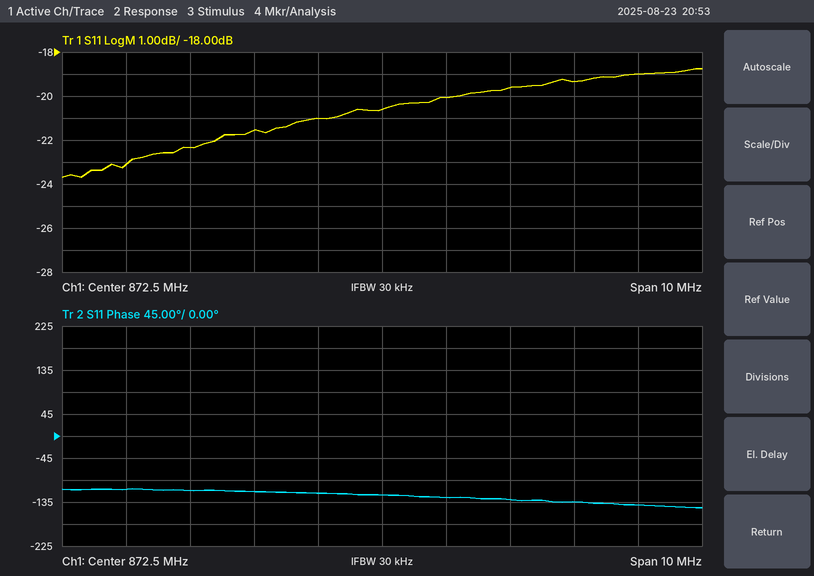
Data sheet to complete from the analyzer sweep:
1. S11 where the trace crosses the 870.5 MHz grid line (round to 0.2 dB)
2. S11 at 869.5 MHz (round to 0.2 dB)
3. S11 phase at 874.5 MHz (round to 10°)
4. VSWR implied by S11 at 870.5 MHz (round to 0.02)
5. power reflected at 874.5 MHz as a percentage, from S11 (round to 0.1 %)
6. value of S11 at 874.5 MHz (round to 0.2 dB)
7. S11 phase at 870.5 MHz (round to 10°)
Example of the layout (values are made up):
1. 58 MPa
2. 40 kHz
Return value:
1. -21.6 dB
2. -22.4 dB
3. -130°
4. 1.18
5. 1.1 %
6. -19.6 dB
7. -110°
